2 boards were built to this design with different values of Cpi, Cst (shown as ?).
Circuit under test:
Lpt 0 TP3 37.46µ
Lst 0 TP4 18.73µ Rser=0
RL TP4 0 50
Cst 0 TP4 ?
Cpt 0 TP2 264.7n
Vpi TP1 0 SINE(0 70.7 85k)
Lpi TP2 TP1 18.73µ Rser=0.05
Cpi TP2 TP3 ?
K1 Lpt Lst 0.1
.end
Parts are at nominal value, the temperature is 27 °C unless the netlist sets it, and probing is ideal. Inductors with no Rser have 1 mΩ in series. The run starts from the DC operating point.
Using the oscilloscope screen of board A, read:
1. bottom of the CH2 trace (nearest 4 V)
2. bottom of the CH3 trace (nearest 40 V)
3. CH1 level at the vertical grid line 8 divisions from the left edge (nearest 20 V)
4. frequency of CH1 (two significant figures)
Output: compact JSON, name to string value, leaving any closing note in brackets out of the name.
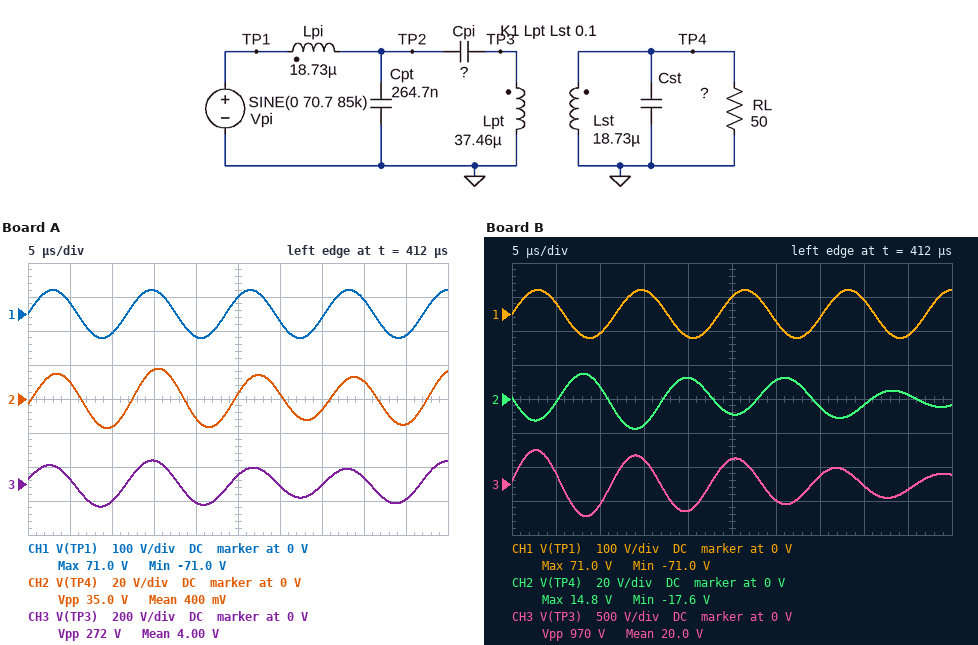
{"bottom of the CH2 trace": "-16 V", "bottom of the CH3 trace": "-120 V", "CH1 level at the vertical grid line 8 divisions from the left edge": "40 V", "frequency of CH1": "85 kHz"}
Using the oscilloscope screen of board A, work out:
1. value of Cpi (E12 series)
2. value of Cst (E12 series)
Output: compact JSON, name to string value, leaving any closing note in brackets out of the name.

{"value of Cpi": "68 nF", "value of Cst": "100 nF"}
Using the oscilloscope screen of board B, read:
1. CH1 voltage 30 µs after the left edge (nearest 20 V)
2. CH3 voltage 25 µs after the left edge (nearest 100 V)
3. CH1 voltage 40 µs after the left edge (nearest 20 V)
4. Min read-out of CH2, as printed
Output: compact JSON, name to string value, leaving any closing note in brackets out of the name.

{"CH1 voltage 30 µs after the left edge": "-20 V", "CH3 voltage 25 µs after the left edge": "400 V", "CH1 voltage 40 µs after the left edge": "40 V", "Min read-out of CH2, as printed": "-17.6 V"}
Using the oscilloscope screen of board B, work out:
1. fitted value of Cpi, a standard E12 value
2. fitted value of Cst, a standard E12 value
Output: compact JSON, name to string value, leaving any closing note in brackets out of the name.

{"fitted value of Cpi, a standard E12 value": "270 nF", "fitted value of Cst, a standard E12 value": "560 nF"}
